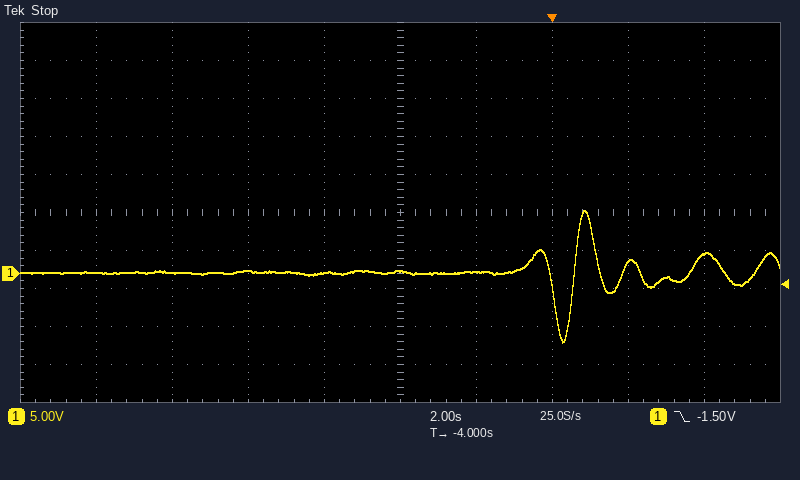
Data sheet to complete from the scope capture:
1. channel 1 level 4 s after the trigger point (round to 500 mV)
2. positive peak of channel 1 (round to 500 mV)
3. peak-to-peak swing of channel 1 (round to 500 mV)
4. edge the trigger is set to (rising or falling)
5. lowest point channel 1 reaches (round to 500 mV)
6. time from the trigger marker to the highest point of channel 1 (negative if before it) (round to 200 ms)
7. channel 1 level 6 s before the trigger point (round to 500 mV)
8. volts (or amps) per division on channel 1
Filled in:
2.5 V
8.5 V
17.5 V
falling
-9.0 V
+800 ms
0.0 V
5 V
